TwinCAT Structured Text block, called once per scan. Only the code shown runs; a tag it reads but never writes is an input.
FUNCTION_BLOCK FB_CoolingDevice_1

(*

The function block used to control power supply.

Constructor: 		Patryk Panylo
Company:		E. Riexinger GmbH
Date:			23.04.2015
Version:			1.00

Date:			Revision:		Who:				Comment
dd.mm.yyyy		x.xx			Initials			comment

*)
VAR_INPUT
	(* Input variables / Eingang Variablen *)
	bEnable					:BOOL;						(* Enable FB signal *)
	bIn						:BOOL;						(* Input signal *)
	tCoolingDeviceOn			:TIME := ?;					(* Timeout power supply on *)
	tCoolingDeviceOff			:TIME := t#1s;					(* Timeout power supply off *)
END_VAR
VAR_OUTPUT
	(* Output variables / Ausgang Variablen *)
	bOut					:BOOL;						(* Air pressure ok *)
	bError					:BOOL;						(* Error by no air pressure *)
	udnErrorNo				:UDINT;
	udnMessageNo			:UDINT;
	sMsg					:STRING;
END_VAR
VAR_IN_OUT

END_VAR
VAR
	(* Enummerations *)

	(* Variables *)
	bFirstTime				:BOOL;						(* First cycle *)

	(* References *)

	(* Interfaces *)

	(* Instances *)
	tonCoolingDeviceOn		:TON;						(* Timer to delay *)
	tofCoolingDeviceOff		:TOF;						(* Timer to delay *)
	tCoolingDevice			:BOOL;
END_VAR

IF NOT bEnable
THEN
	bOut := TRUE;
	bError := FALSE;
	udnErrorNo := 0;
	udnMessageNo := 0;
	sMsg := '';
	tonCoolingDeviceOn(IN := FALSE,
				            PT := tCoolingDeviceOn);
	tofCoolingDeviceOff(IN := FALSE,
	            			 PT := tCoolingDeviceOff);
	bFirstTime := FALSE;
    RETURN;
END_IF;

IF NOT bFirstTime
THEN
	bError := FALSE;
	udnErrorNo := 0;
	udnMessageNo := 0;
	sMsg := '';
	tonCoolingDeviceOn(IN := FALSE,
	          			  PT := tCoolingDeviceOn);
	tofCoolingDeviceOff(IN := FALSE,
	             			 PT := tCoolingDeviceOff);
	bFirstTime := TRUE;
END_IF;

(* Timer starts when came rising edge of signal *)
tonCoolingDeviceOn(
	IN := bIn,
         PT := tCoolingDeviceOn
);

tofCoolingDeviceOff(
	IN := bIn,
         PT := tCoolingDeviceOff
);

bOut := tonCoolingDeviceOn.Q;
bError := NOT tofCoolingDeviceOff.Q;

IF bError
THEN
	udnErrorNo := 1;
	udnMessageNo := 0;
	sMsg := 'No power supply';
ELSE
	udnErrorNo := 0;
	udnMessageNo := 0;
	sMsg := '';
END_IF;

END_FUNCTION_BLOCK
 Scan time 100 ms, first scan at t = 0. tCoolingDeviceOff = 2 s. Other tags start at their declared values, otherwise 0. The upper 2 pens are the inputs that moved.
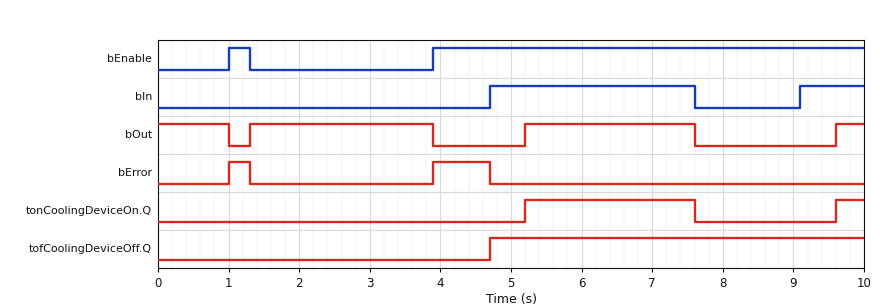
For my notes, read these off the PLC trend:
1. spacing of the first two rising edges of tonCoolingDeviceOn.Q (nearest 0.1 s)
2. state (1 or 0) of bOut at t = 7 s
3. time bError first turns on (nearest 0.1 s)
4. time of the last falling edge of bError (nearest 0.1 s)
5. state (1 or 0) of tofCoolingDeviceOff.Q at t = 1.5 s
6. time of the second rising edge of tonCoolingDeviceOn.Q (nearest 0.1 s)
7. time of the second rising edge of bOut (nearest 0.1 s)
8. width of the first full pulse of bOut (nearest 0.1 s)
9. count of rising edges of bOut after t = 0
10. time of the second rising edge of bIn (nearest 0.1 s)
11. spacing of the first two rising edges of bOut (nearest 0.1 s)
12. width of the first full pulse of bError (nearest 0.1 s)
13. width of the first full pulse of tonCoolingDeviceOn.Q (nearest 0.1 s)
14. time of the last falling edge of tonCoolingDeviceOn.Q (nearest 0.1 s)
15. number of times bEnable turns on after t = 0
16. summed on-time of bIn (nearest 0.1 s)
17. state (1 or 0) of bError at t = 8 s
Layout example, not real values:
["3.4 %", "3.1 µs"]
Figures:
["4.4 s", "1", "1.0 s", "4.7 s", "0", "9.6 s", "5.2 s", "2.6 s", "3", "9.1 s", "3.9 s", "0.3 s", "2.4 s", "7.6 s", "2", "3.8 s", "0"]
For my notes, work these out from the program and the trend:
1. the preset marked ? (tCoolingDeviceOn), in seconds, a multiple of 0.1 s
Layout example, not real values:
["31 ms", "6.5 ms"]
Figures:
["0.5 s"]
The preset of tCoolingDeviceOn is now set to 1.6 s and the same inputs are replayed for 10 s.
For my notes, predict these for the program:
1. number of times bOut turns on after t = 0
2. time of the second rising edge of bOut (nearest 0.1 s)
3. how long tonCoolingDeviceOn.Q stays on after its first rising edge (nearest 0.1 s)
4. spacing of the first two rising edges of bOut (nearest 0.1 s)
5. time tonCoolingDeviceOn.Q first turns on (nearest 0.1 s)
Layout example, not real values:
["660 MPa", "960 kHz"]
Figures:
["2", "6.3 s", "1.3 s", "5.0 s", "6.3 s"]
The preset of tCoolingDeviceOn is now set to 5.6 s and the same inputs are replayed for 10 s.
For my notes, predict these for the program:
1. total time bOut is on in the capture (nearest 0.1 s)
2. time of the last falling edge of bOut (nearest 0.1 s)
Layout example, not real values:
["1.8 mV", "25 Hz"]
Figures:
["3.6 s", "3.9 s"]
